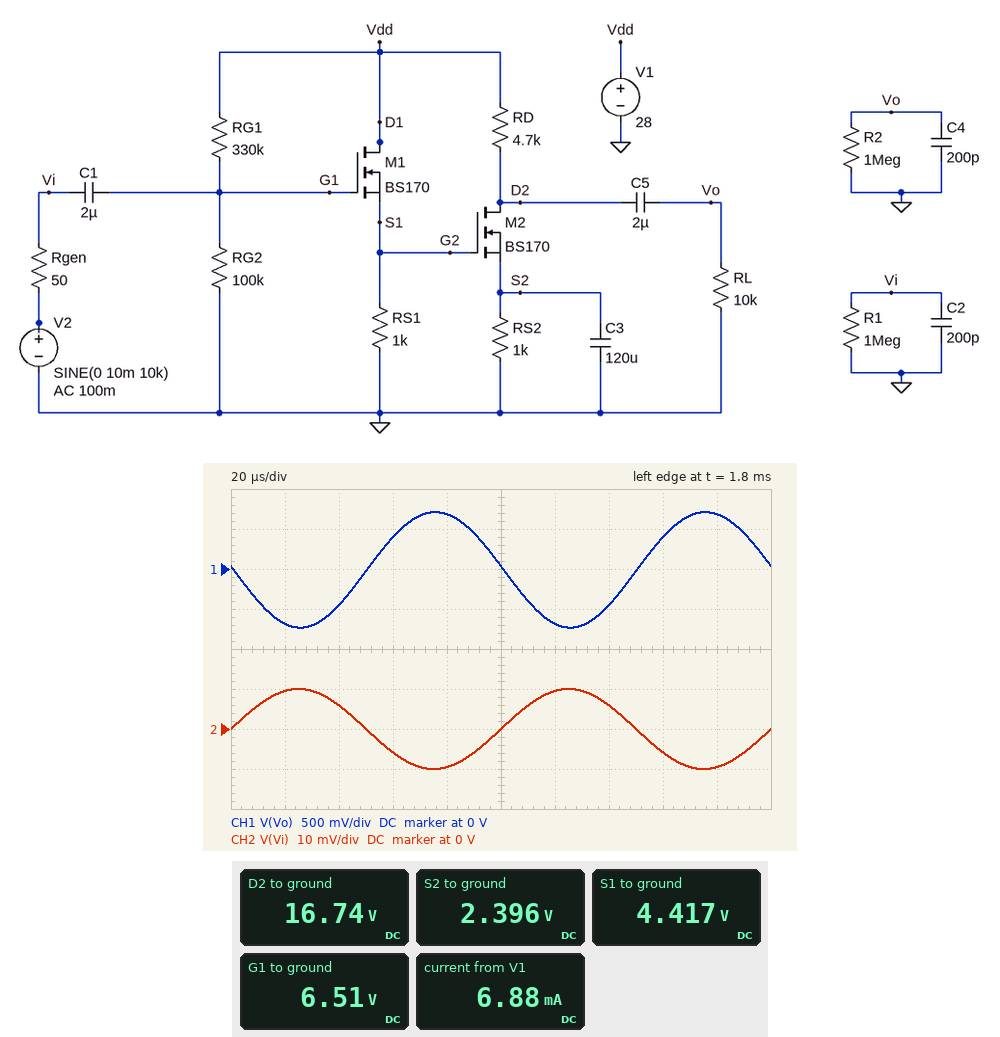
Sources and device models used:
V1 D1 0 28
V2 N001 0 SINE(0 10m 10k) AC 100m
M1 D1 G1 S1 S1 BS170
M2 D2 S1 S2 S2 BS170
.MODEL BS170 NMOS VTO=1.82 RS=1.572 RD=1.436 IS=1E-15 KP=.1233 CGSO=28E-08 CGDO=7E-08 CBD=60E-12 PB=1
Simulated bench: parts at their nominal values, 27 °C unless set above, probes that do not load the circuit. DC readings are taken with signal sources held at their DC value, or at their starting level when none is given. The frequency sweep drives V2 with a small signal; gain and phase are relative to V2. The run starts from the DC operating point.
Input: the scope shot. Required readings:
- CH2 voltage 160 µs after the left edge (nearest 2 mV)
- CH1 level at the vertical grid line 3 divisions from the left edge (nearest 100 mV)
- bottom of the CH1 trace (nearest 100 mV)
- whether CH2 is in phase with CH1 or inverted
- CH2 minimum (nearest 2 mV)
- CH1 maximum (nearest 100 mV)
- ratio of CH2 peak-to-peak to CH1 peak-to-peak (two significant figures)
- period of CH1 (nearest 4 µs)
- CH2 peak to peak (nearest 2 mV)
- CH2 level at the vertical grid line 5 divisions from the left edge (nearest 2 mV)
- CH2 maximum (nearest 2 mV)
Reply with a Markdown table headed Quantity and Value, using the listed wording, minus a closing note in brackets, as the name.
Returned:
| Quantity | Value |
|---|---|
| CH2 voltage 160 µs after the left edge | -6 mV |
| CH1 level at the vertical grid line 3 divisions from the left edge | 400 mV |
| bottom of the CH1 trace | -700 mV |
| whether CH2 is in phase with CH1 or inverted | inverted |
| CH2 minimum | -10 mV |
| CH1 maximum | 700 mV |
| ratio of CH2 peak-to-peak to CH1 peak-to-peak | 0.014 |
| period of CH1 | 100 µs |
| CH2 peak to peak | 20 mV |
| CH2 level at the vertical grid line 5 divisions from the left edge | 0 V |
| CH2 maximum | 10 mV |
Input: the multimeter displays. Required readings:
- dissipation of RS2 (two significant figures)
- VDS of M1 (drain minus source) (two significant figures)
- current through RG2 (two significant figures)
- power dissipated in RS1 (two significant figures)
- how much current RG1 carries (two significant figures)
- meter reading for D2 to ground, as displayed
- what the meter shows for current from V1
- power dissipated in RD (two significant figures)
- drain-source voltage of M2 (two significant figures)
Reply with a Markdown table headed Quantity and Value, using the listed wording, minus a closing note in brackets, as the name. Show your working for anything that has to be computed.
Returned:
| Quantity | Value |
|---|---|
| dissipation of RS2 | (2.396 V)^2 / 1 kΩ = 5.7 mW |
| VDS of M1 (drain minus source) | 28 V - 4.417 V = 24 V |
| current through RG2 | (6.51 V) / 100 kΩ = 65 µA |
| power dissipated in RS1 | (4.417 V)^2 / 1 kΩ = 20 mW |
| how much current RG1 carries | (28 V - 6.51 V) / 330 kΩ = 65 µA |
| meter reading for D2 to ground, as displayed | 16.74 V |
| what the meter shows for current from V1 | 6.88 mA |
| power dissipated in RD | (28 V - 16.74 V)^2 / 4.7 kΩ = 27 mW |
| drain-source voltage of M2 | 16.74 V - 2.396 V = 14 V |
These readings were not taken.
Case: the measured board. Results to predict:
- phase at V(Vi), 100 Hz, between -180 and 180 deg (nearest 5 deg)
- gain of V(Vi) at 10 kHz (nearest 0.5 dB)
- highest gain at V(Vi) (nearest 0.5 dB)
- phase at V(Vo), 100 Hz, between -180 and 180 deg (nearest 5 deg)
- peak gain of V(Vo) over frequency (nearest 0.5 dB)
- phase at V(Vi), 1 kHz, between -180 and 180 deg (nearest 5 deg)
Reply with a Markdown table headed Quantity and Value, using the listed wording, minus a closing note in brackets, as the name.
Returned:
| Quantity | Value |
|---|---|
| phase at V(Vi), 100 Hz, between -180 and 180 deg | 0 deg |
| gain of V(Vi) at 10 kHz | 0 dB |
| highest gain at V(Vi) | 0 dB |
| phase at V(Vo), 100 Hz, between -180 and 180 deg | -160 deg |
| peak gain of V(Vo) over frequency | 37.0 dB |
| phase at V(Vi), 1 kHz, between -180 and 180 deg | 0 deg |
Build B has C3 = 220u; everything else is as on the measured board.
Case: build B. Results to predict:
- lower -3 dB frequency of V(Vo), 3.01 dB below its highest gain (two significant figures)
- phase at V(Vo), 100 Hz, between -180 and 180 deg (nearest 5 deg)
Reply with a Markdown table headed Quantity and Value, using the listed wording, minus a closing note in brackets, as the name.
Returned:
| Quantity | Value |
|---|---|
| lower -3 dB frequency of V(Vo), 3.01 dB below its highest gain | 19 Hz |
| phase at V(Vo), 100 Hz, between -180 and 180 deg | -165 deg |
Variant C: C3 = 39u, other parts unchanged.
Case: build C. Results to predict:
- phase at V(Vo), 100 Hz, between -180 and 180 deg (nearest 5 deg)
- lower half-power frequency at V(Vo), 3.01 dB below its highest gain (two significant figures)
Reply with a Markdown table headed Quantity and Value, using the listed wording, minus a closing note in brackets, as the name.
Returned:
| Quantity | Value |
|---|---|
| phase at V(Vo), 100 Hz, between -180 and 180 deg | -135 deg |
| lower half-power frequency at V(Vo), 3.01 dB below its highest gain | 100 Hz |
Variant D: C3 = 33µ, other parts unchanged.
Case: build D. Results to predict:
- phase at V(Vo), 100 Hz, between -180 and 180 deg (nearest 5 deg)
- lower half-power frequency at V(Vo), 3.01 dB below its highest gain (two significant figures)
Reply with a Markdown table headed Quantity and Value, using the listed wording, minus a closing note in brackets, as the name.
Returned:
| Quantity | Value |
|---|---|
| phase at V(Vo), 100 Hz, between -180 and 180 deg | -130 deg |
| lower half-power frequency at V(Vo), 3.01 dB below its highest gain | 120 Hz |
